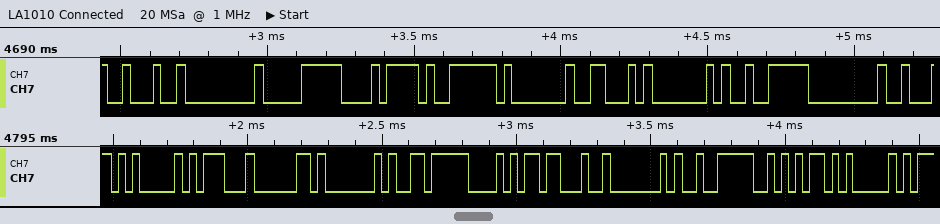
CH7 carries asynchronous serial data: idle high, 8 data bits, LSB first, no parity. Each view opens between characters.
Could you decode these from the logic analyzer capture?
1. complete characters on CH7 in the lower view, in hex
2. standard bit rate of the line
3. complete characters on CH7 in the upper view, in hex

05, 1D, 60, 40, F6, A8, 23, 40, F2, AA, 05
38400 baud
22, 00, F0, E8, F9, 01, 46, 40, F2, 00
